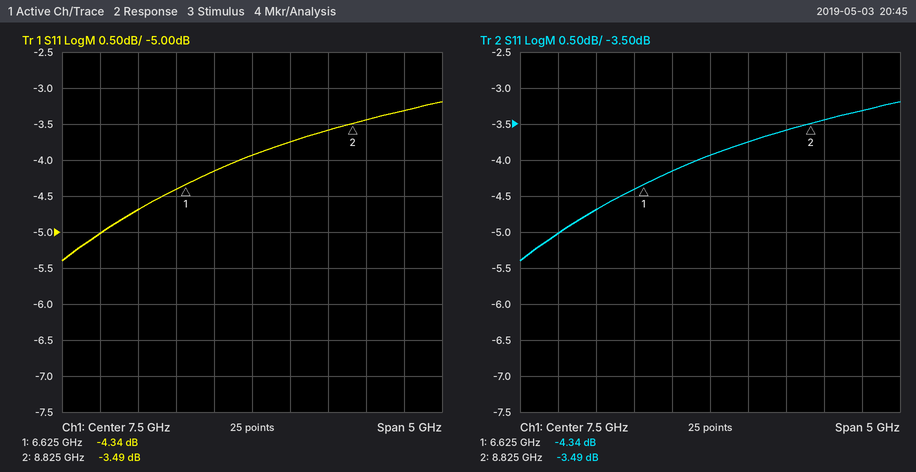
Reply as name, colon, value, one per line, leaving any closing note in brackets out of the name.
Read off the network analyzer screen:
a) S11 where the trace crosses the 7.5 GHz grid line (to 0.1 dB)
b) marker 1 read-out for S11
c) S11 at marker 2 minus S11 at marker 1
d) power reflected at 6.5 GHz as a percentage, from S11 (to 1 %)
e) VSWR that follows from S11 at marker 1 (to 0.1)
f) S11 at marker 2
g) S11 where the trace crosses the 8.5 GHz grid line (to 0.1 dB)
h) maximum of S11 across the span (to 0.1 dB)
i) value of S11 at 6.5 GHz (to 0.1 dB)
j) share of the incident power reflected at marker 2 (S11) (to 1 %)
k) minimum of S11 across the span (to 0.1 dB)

S11 where the trace crosses the 7.5 GHz grid line: -3.9 dB
marker 1 read-out for S11: -4.34 dB
S11 at marker 2 minus S11 at marker 1: 0.85 dB
power reflected at 6.5 GHz as a percentage, from S11: 36 %
VSWR that follows from S11 at marker 1: 4.1
S11 at marker 2: -3.49 dB
S11 where the trace crosses the 8.5 GHz grid line: -3.6 dB
maximum of S11 across the span: -3.2 dB
value of S11 at 6.5 GHz: -4.4 dB
share of the incident power reflected at marker 2 (S11): 45 %
minimum of S11 across the span: -5.4 dB
